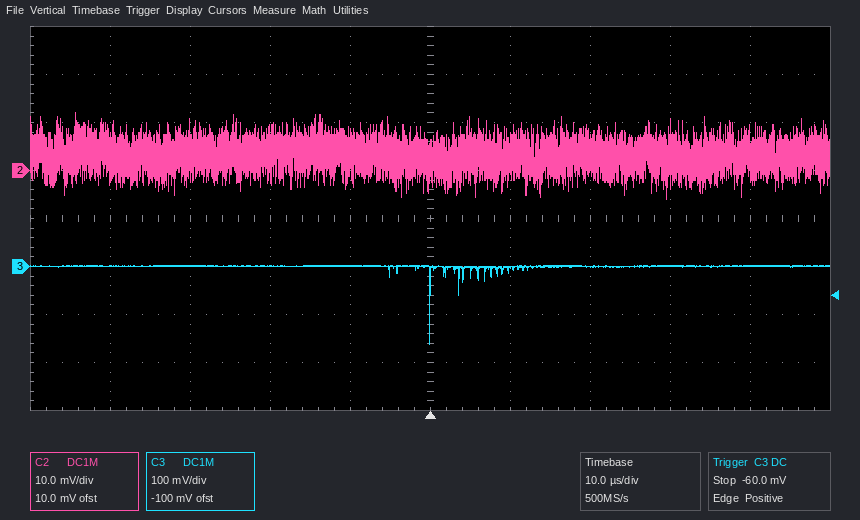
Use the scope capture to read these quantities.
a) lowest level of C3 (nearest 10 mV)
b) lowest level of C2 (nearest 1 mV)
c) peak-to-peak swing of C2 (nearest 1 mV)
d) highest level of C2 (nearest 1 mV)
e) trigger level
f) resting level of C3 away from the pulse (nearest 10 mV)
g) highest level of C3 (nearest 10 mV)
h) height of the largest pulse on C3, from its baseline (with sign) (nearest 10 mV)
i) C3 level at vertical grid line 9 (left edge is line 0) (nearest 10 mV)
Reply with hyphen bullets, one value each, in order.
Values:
- -160 mV
- -6 mV
- 18 mV
- 12 mV
- -60.0 mV
- 0 mV
- 0 mV
- -160 mV
- 0 mV
